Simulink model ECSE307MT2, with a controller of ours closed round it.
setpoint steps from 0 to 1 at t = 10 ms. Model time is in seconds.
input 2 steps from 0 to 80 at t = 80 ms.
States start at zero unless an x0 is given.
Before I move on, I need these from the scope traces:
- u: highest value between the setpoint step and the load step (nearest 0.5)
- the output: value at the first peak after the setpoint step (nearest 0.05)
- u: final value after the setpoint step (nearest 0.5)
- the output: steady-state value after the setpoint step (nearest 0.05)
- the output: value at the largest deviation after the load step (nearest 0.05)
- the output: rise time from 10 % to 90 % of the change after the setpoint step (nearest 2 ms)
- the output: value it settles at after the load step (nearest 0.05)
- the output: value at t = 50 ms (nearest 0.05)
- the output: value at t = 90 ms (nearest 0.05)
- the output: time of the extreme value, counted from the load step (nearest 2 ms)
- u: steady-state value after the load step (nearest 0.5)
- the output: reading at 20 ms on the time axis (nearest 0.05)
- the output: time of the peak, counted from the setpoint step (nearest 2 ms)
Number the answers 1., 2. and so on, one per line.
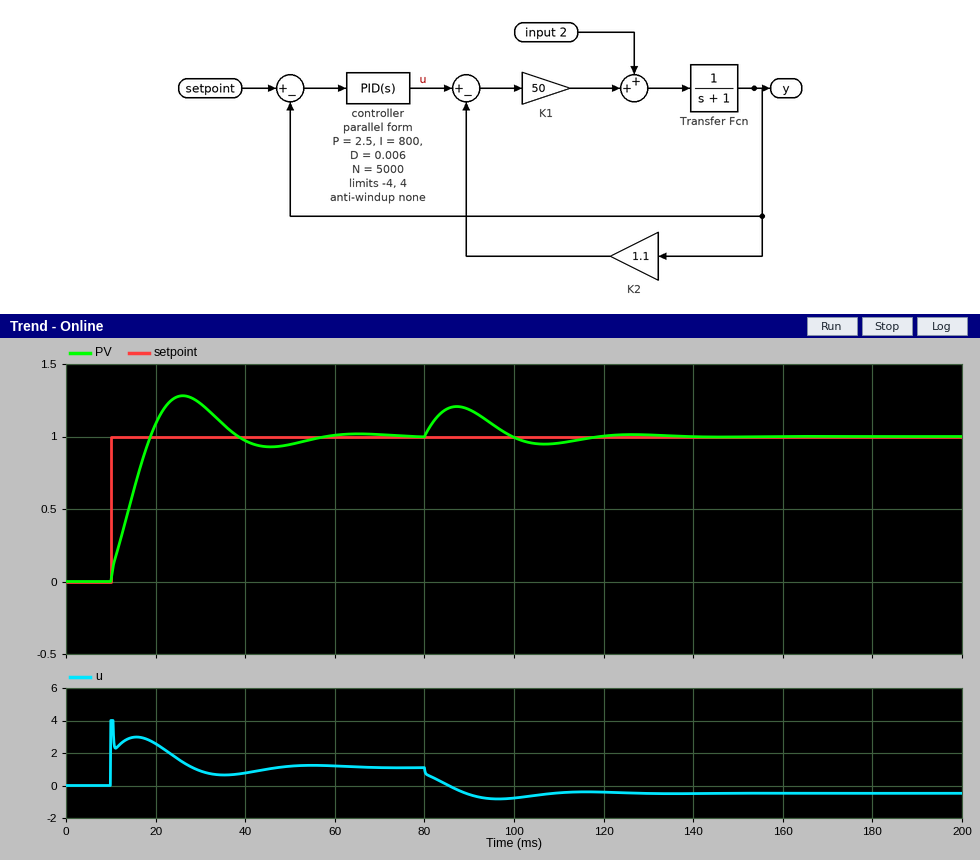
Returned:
1. 4.0
2. 1.30
3. 1.0
4. 1.00
5. 1.20
6. 8 ms
7. 1.00
8. 0.95
9. 1.20
10. 8 ms
11. -0.5
12. 1.10
13. 16 ms
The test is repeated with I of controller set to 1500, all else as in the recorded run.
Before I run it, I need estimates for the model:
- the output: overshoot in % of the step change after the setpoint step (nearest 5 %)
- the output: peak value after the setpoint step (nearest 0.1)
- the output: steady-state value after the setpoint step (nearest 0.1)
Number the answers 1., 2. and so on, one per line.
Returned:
1. 40 %
2. 1.4
3. 1.0
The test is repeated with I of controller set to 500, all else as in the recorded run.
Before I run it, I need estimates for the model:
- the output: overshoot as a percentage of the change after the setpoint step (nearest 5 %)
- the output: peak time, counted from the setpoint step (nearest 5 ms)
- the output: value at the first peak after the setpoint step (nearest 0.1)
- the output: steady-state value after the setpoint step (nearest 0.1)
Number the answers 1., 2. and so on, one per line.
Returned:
1. 20 %
2. 20 ms
3. 1.2
4. 1.0
